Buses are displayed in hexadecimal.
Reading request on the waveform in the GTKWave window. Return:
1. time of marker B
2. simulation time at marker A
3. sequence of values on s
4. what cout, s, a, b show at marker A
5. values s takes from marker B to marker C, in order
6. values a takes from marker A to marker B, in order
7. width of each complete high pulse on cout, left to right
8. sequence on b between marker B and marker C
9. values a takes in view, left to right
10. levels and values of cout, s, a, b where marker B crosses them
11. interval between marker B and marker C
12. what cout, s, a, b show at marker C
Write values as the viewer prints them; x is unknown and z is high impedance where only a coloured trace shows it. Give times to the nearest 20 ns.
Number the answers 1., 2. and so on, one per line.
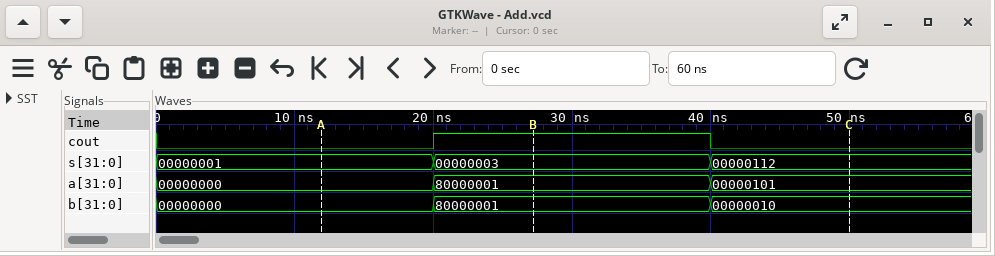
1. 20 ns
2. 20 ns
3. 00000001, 00000003, 00000112
4. cout=0, s=00000001, a=00000000, b=00000000
5. 00000003, 00000112
6. 00000000, 80000001
7. 20 ns
8. 80000001, 00000010
9. 00000000, 80000001, 00000101
10. cout=1, s=00000003, a=80000001, b=80000001
11. 20 ns
12. cout=0, s=00000112, a=00000101, b=00000010
